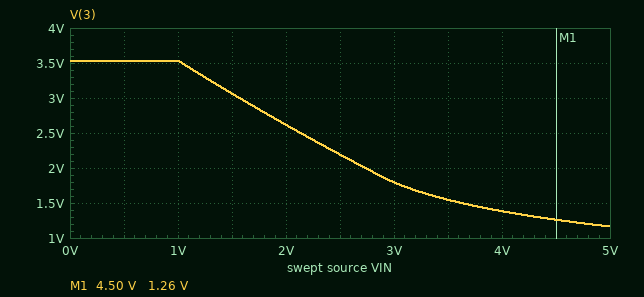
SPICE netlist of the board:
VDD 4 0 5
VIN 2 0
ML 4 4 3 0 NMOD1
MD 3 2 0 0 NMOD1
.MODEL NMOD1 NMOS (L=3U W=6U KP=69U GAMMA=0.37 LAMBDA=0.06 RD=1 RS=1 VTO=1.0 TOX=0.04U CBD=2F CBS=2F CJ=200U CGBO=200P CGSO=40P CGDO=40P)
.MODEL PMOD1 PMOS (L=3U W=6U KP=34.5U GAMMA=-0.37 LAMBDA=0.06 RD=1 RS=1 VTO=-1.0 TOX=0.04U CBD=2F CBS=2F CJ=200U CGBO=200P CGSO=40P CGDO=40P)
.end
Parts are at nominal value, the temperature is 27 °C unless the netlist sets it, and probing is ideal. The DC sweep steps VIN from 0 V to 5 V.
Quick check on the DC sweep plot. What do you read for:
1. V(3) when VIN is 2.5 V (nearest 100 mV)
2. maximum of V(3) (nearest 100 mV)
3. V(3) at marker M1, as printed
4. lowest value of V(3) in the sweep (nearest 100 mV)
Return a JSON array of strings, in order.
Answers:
["2.2 V", "3.5 V", "1.26 V", "1.2 V"]
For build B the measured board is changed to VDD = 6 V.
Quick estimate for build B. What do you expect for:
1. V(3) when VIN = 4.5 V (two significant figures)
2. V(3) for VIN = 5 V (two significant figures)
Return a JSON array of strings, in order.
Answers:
["1.8 V", "1.7 V"]
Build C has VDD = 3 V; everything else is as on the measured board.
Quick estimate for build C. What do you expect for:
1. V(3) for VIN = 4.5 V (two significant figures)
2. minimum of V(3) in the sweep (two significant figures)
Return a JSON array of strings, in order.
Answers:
["400 mV", "360 mV"]
